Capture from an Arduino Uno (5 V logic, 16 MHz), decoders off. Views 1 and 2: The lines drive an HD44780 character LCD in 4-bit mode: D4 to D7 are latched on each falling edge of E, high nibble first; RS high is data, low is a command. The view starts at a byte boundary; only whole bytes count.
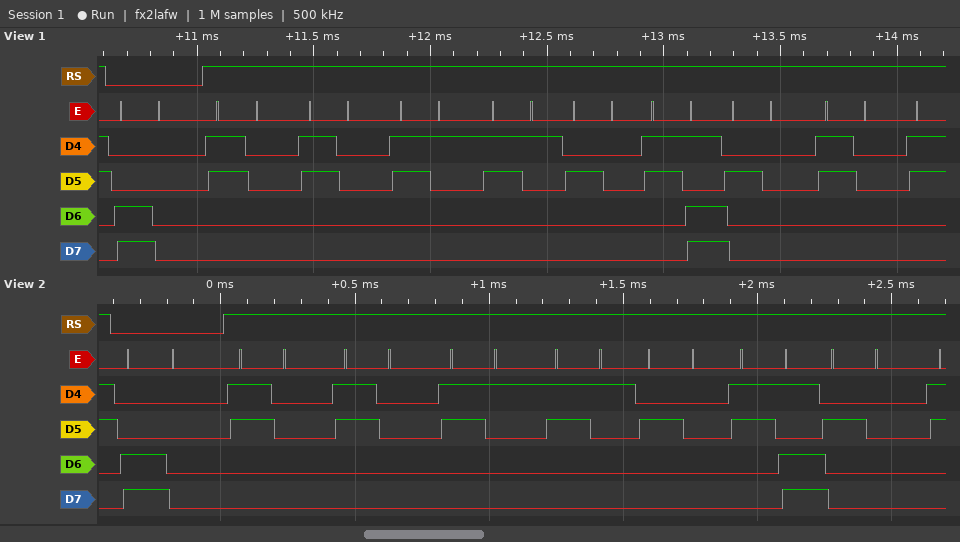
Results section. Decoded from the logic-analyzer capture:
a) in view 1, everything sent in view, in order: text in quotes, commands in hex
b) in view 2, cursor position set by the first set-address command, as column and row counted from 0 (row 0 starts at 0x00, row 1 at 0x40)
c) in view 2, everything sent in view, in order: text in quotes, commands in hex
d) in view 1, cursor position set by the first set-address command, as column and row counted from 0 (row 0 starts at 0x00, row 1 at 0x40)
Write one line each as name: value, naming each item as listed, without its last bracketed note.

in view 1, everything sent in view, in order: text in quotes, commands in hex: 0xC0 "0011 = 0"
in view 2, cursor position set by the first set-address command, as column and row counted from 0: column 0, row 1
in view 2, everything sent in view, in order: text in quotes, commands in hex: 0xC0 "0011 = "
in view 1, cursor position set by the first set-address command, as column and row counted from 0: column 0, row 1
